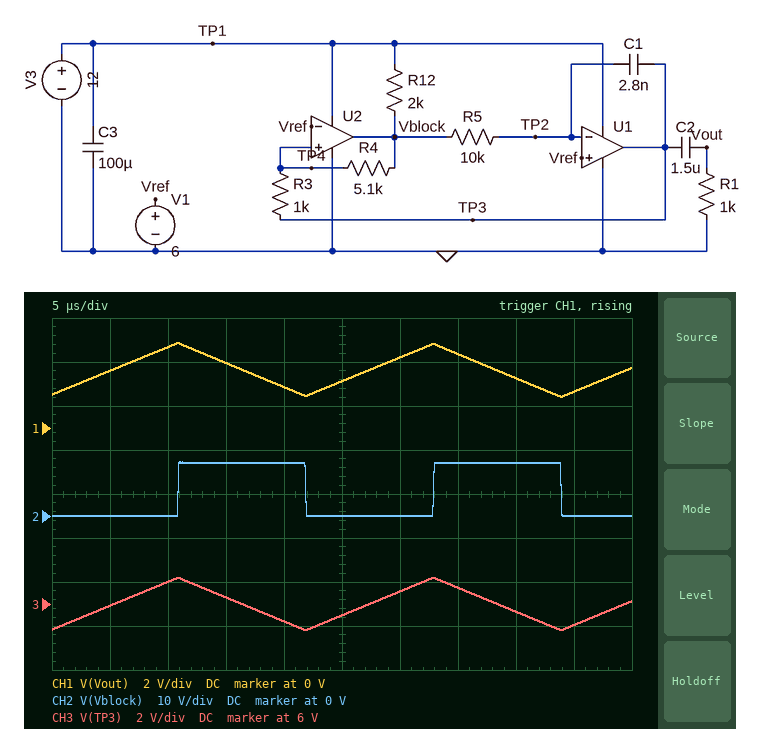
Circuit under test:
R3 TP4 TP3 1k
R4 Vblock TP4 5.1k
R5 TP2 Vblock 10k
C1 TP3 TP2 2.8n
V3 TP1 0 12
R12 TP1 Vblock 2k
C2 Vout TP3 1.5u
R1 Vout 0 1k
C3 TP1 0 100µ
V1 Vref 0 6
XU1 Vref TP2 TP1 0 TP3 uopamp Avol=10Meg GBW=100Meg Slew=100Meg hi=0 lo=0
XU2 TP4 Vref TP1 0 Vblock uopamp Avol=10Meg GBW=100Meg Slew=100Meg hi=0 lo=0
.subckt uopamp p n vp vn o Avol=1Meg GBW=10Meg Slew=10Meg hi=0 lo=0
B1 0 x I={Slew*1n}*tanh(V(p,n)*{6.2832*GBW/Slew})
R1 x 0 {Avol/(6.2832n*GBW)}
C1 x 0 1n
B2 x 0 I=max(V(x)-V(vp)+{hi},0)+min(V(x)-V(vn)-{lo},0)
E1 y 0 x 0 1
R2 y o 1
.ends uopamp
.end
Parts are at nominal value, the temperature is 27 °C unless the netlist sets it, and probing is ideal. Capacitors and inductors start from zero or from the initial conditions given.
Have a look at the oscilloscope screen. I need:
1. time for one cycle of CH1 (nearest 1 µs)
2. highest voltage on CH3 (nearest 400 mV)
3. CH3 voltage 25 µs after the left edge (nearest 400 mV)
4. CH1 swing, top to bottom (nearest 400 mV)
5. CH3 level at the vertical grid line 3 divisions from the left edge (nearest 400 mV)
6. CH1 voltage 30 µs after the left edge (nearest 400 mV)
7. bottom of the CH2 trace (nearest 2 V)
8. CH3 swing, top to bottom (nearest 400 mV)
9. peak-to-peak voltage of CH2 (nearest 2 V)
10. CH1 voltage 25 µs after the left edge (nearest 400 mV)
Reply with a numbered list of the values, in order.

1. 22 µs
2. 7.2 V
3. 5.6 V
4. 2.4 V
5. 6.4 V
6. 3.2 V
7. 0 V
8. 2.4 V
9. 12 V
10. 2.0 V
